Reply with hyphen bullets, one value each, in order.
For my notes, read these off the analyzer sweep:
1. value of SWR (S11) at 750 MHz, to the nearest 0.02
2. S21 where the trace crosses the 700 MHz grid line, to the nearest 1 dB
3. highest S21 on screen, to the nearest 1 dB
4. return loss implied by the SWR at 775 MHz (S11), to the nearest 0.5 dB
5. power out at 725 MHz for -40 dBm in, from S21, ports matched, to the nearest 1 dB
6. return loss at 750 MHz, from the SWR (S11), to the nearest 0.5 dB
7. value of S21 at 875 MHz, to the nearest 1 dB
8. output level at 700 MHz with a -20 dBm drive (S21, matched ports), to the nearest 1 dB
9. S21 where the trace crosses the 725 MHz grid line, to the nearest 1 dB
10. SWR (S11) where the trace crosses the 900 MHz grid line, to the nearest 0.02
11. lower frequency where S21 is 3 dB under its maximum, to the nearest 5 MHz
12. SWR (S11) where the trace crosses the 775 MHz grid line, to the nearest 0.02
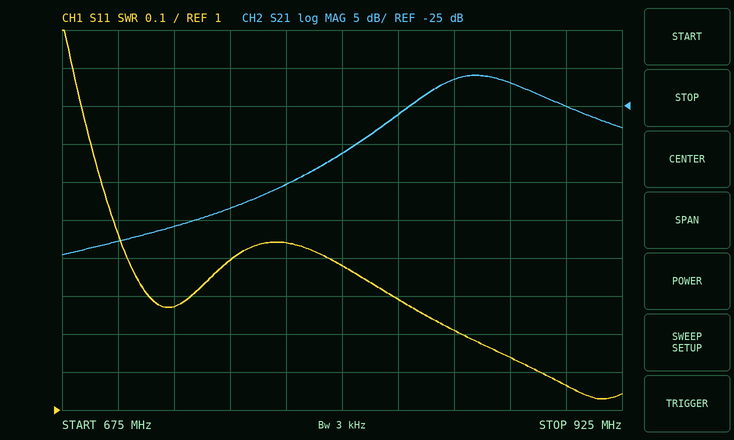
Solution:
- 1.40
- -43 dB
- -21 dB
- 15.0 dB
- -81 dBm
- 15.5 dB
- -22 dB
- -63 dBm
- -41 dB
- 1.06
- 835 MHz
- 1.44
